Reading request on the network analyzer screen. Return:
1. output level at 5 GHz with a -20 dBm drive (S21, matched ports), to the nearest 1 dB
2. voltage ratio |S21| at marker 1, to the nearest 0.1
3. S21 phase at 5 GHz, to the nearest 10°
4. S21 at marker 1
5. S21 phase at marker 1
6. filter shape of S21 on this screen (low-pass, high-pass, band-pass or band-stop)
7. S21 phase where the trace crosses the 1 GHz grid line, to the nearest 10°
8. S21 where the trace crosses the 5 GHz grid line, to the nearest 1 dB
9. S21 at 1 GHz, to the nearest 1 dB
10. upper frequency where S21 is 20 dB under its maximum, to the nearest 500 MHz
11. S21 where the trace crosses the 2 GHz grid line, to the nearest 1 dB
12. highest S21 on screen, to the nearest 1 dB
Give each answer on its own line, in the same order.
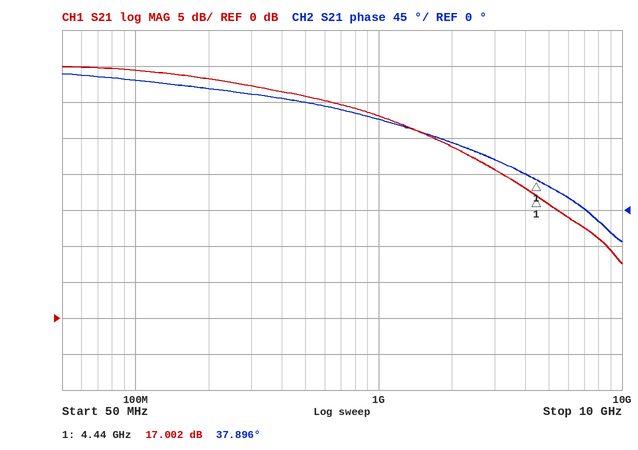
-4 dBm
7.1
30°
17.002 dB
37.896°
low-pass
110°
16 dB
28 dB
5.5 GHz
24 dB
35 dB
